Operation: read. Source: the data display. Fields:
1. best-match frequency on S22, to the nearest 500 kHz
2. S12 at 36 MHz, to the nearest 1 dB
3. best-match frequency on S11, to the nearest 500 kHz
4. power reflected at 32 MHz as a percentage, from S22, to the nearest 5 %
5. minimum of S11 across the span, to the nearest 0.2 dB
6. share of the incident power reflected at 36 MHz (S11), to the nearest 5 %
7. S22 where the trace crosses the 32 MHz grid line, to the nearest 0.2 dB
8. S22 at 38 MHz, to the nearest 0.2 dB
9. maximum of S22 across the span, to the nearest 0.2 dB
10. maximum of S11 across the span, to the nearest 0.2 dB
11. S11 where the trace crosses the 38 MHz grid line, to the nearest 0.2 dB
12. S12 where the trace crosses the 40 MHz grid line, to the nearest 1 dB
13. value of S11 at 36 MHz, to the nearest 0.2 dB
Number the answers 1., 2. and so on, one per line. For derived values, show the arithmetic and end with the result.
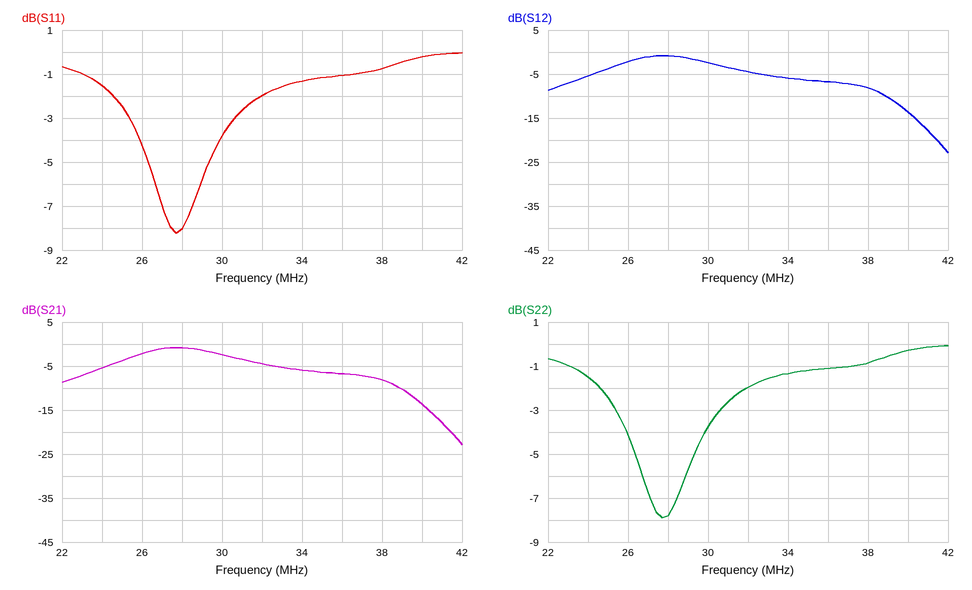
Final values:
1. 27.5 MHz
2. -7 dB
3. 27.5 MHz
4. 10^(-2/10) ≈ 63.1 %, so 65 % to the nearest 5 %
5. -8.2 dB
6. 10^(-1/10) ≈ 79.4 %, so 80 % to the nearest 5 %
7. -2.0 dB
8. -0.8 dB
9. 0.0 dB
10. 0.0 dB
11. -0.8 dB
12. -14 dB
13. -1.0 dB
